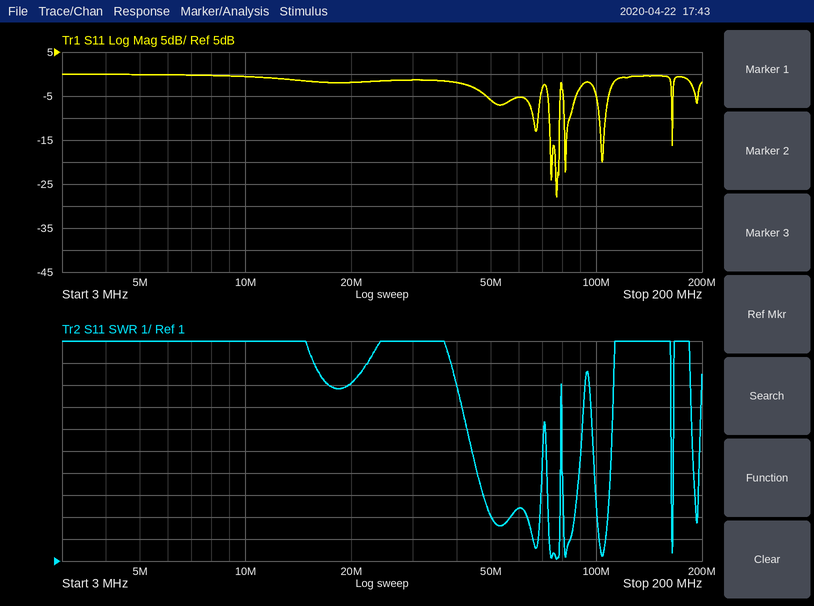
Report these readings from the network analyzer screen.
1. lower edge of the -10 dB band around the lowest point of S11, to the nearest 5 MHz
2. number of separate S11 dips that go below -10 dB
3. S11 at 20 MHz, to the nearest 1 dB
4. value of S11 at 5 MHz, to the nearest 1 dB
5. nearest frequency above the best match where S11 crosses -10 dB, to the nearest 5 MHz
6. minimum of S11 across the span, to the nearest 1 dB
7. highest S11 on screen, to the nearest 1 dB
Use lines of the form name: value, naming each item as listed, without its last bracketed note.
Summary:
lower edge of the -10 dB band around the lowest point of S11, to the nearest 5 MHz: 75 MHz
number of separate S11 dips that go below -10 dB: 6
S11 at 20 MHz, to the nearest 1 dB: -2 dB
value of S11 at 5 MHz, to the nearest 1 dB: 0 dB
nearest frequency above the best match where S11 crosses -10 dB, to the nearest 5 MHz: 80 MHz
minimum of S11 across the span, to the nearest 1 dB: -28 dB
highest S11 on screen, to the nearest 1 dB: 0 dB
